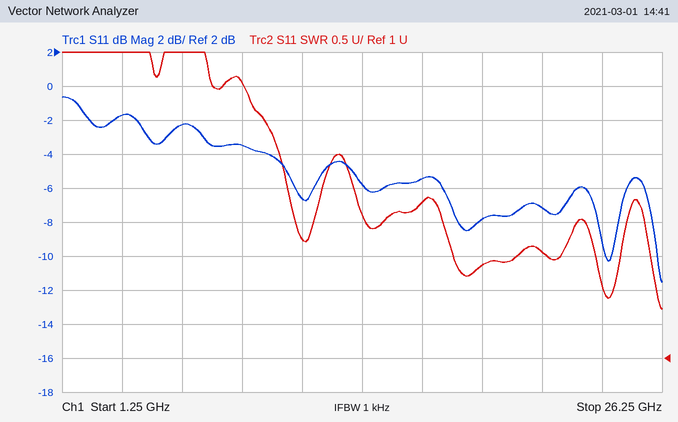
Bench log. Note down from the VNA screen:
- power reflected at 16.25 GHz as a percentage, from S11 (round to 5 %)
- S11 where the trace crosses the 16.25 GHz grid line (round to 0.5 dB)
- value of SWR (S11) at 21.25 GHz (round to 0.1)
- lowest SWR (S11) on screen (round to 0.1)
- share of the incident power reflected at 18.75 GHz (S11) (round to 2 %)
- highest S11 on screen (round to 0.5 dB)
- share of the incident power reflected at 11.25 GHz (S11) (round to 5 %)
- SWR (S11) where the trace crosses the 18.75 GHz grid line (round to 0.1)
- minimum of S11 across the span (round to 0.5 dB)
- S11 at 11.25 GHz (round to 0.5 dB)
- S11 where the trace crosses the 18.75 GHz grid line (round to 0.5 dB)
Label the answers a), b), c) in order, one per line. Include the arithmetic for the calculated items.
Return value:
a) 10^(-5.5/10) ≈ 28.2 %, so 30 % to the nearest 5 %
b) -5.5 dB
c) 2.6
d) 1.7
e) 10^(-8/10) ≈ 16 %
f) -0.5 dB
g) 10^(-6.5/10) ≈ 22.4 %, so 20 % to the nearest 5 %
h) 2.4
i) -11.5 dB
j) -6.5 dB
k) -8.0 dB
